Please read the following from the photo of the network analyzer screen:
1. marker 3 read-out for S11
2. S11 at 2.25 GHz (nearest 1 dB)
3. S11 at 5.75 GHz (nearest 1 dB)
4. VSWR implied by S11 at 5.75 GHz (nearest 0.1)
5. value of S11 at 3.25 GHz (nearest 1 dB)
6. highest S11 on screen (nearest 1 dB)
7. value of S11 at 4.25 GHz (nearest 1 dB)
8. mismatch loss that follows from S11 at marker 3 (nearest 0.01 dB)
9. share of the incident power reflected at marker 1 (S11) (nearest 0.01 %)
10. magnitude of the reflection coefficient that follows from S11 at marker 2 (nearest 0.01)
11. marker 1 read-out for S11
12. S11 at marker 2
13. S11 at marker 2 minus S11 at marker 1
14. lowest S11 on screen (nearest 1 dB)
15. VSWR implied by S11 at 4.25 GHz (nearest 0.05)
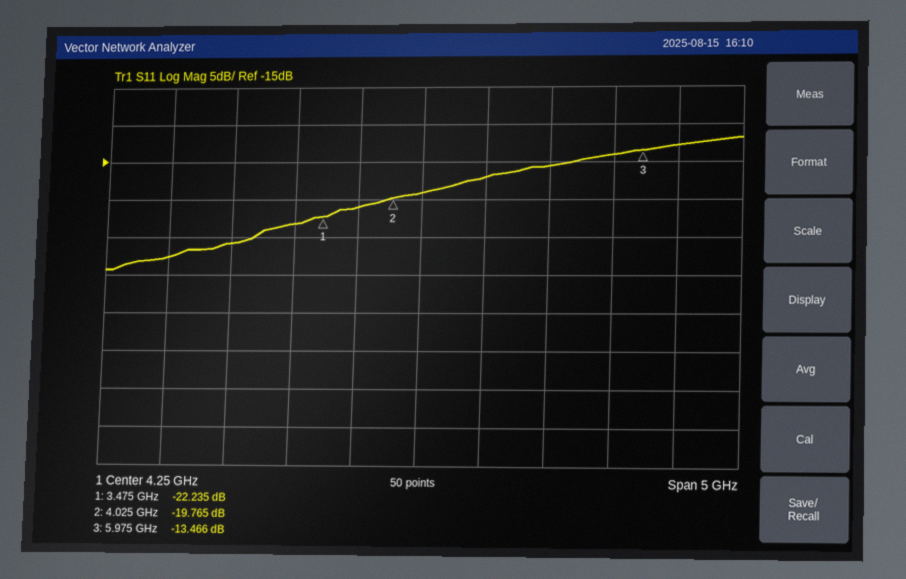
-13.466 dB
-28 dB
-14 dB
1.5
-23 dB
-12 dB
-19 dB
0.20 dB
0.60 %
0.10
-22.235 dB
-19.765 dB
2.470 dB
-29 dB
1.25
